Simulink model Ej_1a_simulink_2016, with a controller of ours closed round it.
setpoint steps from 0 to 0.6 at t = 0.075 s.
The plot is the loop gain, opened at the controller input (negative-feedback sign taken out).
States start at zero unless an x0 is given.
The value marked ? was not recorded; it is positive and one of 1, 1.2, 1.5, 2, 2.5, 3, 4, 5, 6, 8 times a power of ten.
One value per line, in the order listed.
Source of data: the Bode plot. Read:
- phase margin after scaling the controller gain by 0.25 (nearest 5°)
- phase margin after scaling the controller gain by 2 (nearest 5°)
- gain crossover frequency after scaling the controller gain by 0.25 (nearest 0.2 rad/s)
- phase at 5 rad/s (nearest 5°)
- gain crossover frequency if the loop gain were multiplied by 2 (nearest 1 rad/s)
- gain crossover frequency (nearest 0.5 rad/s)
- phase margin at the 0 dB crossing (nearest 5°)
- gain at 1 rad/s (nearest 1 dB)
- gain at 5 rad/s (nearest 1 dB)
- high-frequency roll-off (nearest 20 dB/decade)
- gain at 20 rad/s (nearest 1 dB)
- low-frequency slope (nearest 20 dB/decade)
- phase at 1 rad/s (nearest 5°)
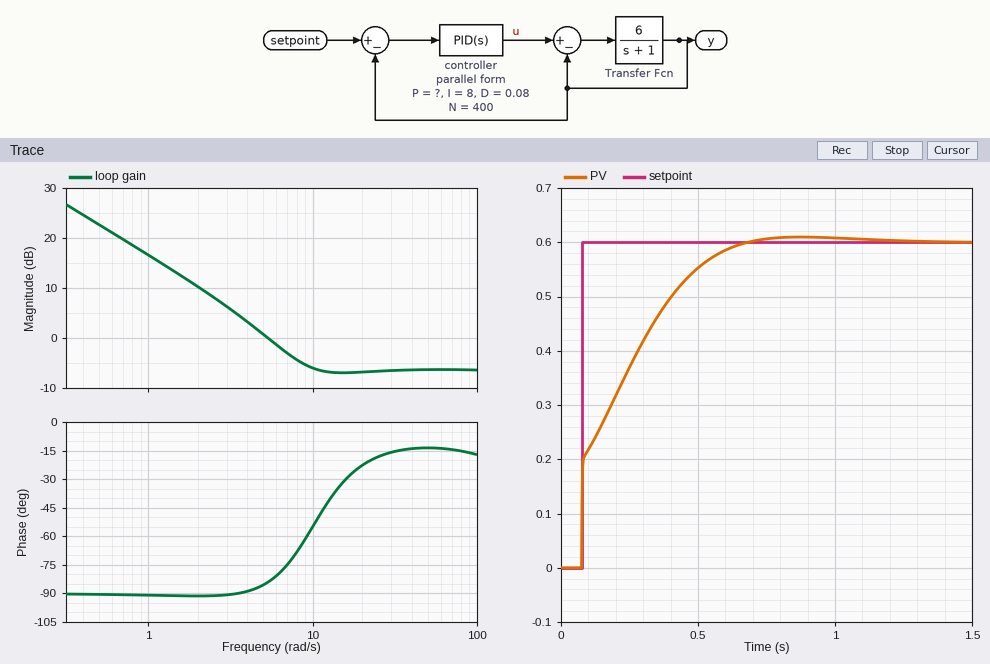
90°
125°
1.6 rad/s
-85°
10 rad/s
5.5 rad/s
95°
17 dB
1 dB
0 dB/decade
-7 dB
-20 dB/decade
-90°
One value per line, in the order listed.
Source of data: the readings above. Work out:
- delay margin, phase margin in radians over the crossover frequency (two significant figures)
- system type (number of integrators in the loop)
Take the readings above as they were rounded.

0.30 s
1
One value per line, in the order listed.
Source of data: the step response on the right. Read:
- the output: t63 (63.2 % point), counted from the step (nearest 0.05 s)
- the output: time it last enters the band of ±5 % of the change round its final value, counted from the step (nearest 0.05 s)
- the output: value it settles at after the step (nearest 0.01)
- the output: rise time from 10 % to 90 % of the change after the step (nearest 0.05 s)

0.20 s
0.45 s
0.60
0.40 s
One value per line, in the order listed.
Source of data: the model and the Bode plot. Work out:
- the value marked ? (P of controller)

1
